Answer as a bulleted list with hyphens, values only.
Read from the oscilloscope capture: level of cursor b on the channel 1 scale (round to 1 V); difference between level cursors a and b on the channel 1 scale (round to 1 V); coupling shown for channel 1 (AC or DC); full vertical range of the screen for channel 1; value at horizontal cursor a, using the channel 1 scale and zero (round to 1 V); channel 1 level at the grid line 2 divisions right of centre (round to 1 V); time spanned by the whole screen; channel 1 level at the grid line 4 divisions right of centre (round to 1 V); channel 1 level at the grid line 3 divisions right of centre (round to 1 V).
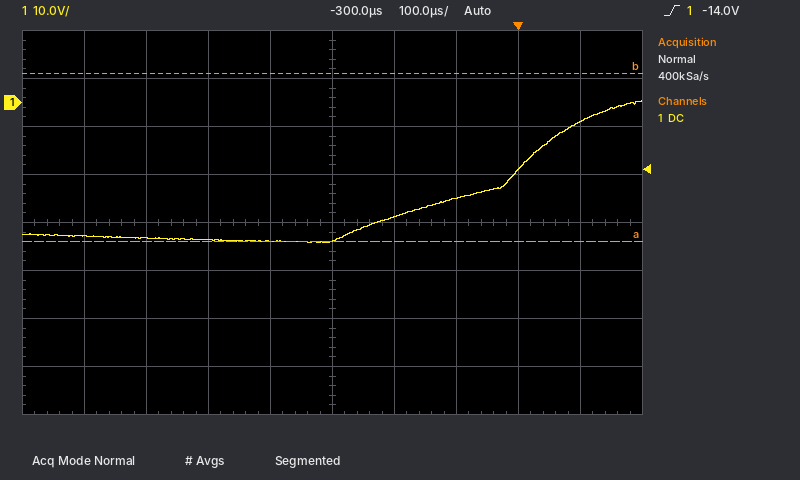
- 6 V
- 35 V
- DC
- 80 V
- -29 V
- -20 V
- 1 ms
- -4 V
- -14 V
